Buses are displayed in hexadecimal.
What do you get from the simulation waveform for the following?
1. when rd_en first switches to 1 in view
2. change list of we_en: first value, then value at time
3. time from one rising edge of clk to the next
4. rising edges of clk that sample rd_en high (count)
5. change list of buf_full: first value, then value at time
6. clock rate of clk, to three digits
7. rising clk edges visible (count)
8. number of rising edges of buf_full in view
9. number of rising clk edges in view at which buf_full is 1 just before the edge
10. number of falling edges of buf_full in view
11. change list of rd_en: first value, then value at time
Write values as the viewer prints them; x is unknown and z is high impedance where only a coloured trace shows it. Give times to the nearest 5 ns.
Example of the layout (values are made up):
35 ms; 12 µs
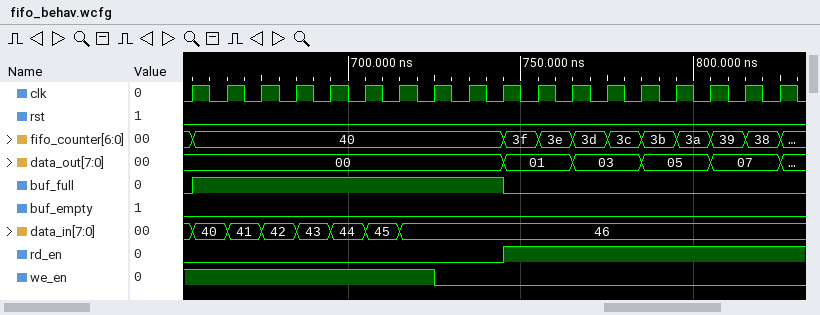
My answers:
745 ns; 1, 0 at 725 ns; 10 ns; 8; 0, 1 at 655 ns, 0 at 745 ns; 100 MHz; 18; 1; 9; 1; 0, 1 at 745 ns
